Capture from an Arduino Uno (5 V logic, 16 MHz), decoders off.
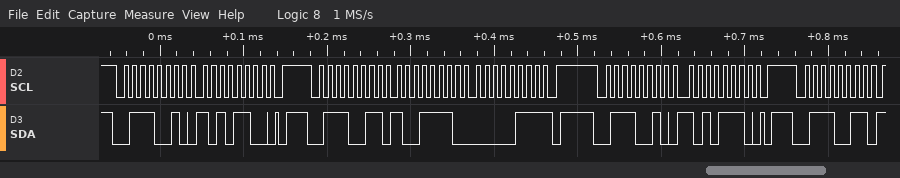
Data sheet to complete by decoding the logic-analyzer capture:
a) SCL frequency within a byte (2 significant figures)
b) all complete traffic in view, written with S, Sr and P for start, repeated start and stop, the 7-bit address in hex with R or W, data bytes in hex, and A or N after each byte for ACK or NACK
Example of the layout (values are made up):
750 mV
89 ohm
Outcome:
100 kHz
S 39W A AC A P S 39R A 9E A 07 N P S 39W A AE A P S 39R A
